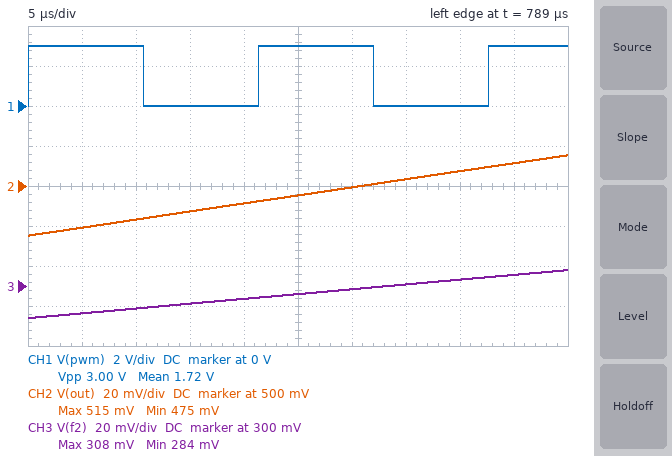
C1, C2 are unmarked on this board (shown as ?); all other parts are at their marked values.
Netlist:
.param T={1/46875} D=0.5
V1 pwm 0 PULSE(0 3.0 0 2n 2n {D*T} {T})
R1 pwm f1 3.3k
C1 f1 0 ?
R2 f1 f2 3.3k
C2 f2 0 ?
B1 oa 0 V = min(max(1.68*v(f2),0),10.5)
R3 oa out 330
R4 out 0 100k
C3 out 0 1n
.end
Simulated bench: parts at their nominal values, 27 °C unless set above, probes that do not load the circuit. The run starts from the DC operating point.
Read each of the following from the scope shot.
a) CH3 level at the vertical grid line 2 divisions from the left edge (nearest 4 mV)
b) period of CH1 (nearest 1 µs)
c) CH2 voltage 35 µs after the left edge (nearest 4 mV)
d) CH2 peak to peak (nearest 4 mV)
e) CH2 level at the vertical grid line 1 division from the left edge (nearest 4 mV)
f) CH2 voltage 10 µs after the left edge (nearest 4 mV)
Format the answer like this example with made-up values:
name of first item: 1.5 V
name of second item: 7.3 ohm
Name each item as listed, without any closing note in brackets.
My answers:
CH3 level at the vertical grid line 2 divisions from the left edge: 288 mV
period of CH1: 21 µs
CH2 voltage 35 µs after the left edge: 504 mV
CH2 peak to peak: 40 mV
CH2 level at the vertical grid line 1 division from the left edge: 480 mV
CH2 voltage 10 µs after the left edge: 484 mV
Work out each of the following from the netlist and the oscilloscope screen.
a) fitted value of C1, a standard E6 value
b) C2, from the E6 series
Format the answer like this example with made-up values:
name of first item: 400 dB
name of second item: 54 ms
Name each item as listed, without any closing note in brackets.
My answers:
fitted value of C1, a standard E6 value: 330 nF
C2, from the E6 series: 220 nF
